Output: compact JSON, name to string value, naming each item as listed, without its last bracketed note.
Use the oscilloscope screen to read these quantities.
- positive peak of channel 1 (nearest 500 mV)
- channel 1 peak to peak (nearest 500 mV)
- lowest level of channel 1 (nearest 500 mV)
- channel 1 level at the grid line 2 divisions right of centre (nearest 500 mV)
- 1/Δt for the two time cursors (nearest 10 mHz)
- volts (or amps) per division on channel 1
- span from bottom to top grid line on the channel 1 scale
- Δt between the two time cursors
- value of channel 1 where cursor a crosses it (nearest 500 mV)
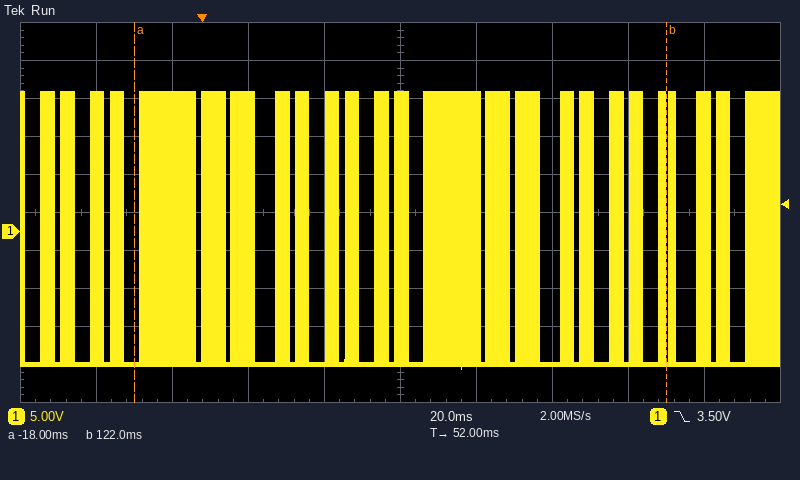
{"positive peak of channel 1": "18.5 V", "channel 1 peak to peak": "36.5 V", "lowest level of channel 1": "-18.0 V", "channel 1 level at the grid line 2 divisions right of centre": "-17.5 V", "1/Δt for the two time cursors": "7.14 Hz", "volts (or amps) per division on channel 1": "5 V", "span from bottom to top grid line on the channel 1 scale": "50 V", "Δt between the two time cursors": "140 ms", "value of channel 1 where cursor a crosses it": "-17.5 V"}
